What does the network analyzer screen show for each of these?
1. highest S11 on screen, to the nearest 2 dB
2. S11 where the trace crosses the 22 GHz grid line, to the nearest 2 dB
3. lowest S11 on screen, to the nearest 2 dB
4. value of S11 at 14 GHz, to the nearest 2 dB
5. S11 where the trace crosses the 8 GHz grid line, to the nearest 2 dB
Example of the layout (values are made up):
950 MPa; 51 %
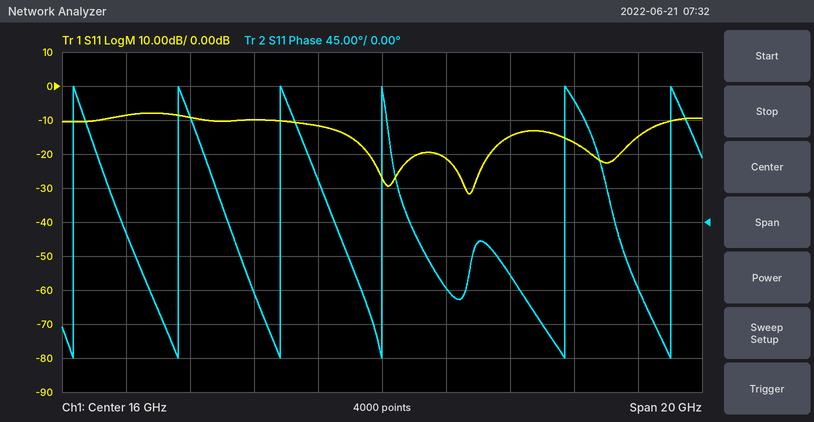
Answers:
-8 dB; -16 dB; -32 dB; -12 dB; -8 dB
